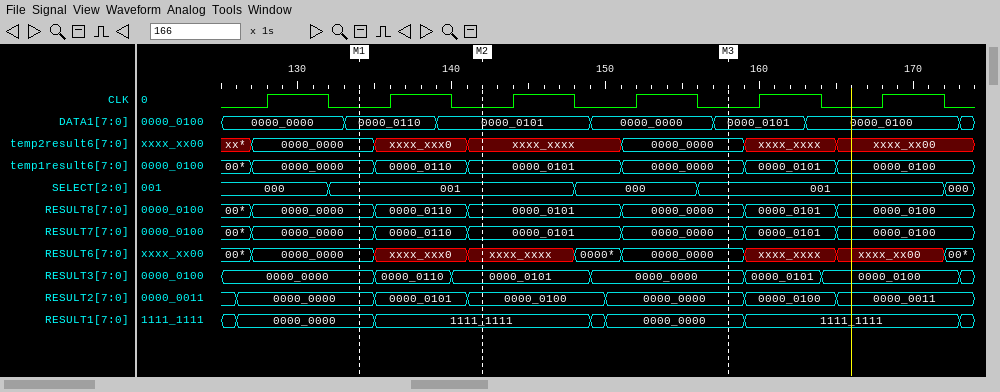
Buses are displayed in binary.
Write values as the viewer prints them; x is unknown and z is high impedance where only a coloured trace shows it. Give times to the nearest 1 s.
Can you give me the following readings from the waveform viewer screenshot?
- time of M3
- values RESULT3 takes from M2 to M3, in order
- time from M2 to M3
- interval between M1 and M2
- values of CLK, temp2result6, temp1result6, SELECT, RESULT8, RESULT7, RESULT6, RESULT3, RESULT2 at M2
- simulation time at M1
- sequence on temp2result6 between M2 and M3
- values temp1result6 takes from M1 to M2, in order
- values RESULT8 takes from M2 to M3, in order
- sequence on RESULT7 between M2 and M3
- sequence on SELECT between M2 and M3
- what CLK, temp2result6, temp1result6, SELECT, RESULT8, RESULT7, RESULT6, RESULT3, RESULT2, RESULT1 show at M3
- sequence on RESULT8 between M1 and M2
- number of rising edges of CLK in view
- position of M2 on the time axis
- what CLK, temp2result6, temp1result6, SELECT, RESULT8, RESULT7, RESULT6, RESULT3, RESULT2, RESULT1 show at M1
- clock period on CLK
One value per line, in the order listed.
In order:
158 s
0000_0101, 0000_0000
16 s
8 s
CLK=0, temp2result6=xxxx_xxxx, temp1result6=0000_0101, SELECT=001, RESULT8=0000_0101, RESULT7=0000_0101, RESULT6=xxxx_xxxx, RESULT3=0000_0101, RESULT2=0000_0100
134 s
xxxx_xxxx, 0000_0000
0000_0000, 0000_0110, 0000_0101
0000_0101, 0000_0000
0000_0101, 0000_0000
001, 000, 001
CLK=0, temp2result6=0000_0000, temp1result6=0000_0000, SELECT=001, RESULT8=0000_0000, RESULT7=0000_0000, RESULT6=0000_0000, RESULT3=0000_0000, RESULT2=0000_0000, RESULT1=0000_0000
0000_0000, 0000_0110, 0000_0101
6
142 s
CLK=0, temp2result6=0000_0000, temp1result6=0000_0000, SELECT=001, RESULT8=0000_0000, RESULT7=0000_0000, RESULT6=0000_0000, RESULT3=0000_0000, RESULT2=0000_0000, RESULT1=0000_0000
8 s
